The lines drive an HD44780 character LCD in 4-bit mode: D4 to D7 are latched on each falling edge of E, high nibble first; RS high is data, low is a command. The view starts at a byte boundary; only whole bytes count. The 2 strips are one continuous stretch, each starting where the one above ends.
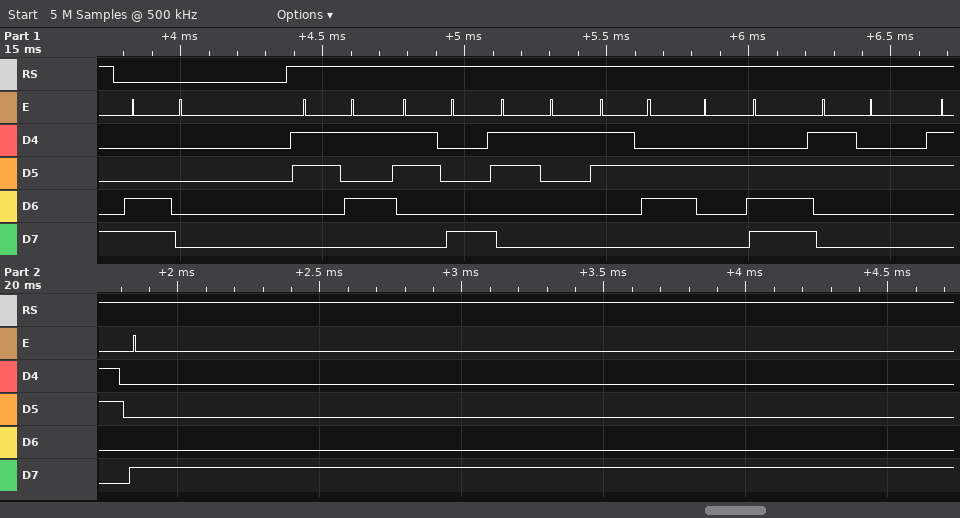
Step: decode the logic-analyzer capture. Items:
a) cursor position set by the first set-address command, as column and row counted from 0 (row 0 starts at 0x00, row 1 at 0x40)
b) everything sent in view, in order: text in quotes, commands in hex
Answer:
column 0, row 1
0xC0 "5816.28"
